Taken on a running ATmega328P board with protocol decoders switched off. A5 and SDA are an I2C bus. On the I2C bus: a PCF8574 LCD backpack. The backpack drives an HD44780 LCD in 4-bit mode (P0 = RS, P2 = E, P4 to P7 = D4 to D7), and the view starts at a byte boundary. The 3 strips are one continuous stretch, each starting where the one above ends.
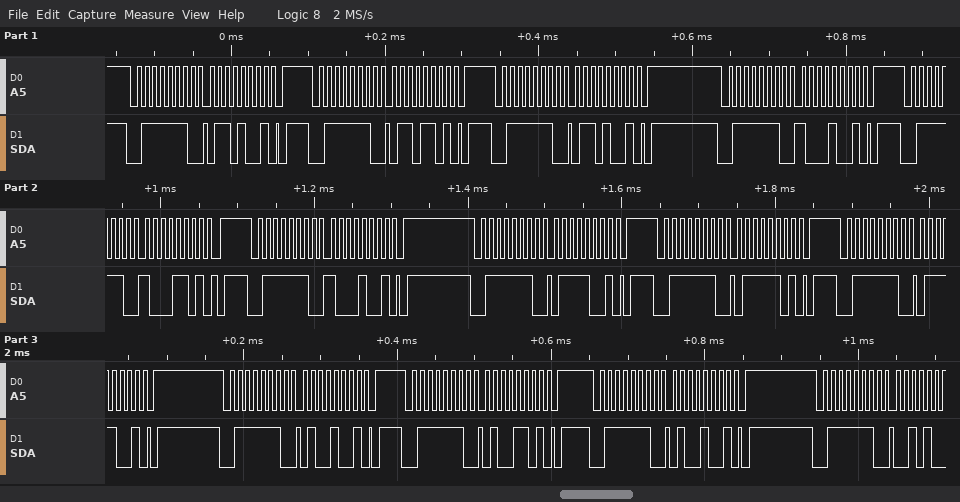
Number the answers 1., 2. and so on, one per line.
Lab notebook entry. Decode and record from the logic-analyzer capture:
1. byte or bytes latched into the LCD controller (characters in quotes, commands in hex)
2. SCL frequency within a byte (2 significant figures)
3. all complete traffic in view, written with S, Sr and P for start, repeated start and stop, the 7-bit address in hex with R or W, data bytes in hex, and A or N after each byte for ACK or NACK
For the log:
1. 'h' 't'
2. 100 kHz
3. S 3FW A 69 A P S 3FW A 6D A P S 3FW A 69 A P S 3FW A 89 A P S 3FW A 8D A P S 3FW A 89 A P S 3FW A 79 A P S 3FW A 7D A P S 3FW A 79 A P S 3FW A 49 A P S 3FW A 4D A P S 3FW A 49 A P S 3FW A
